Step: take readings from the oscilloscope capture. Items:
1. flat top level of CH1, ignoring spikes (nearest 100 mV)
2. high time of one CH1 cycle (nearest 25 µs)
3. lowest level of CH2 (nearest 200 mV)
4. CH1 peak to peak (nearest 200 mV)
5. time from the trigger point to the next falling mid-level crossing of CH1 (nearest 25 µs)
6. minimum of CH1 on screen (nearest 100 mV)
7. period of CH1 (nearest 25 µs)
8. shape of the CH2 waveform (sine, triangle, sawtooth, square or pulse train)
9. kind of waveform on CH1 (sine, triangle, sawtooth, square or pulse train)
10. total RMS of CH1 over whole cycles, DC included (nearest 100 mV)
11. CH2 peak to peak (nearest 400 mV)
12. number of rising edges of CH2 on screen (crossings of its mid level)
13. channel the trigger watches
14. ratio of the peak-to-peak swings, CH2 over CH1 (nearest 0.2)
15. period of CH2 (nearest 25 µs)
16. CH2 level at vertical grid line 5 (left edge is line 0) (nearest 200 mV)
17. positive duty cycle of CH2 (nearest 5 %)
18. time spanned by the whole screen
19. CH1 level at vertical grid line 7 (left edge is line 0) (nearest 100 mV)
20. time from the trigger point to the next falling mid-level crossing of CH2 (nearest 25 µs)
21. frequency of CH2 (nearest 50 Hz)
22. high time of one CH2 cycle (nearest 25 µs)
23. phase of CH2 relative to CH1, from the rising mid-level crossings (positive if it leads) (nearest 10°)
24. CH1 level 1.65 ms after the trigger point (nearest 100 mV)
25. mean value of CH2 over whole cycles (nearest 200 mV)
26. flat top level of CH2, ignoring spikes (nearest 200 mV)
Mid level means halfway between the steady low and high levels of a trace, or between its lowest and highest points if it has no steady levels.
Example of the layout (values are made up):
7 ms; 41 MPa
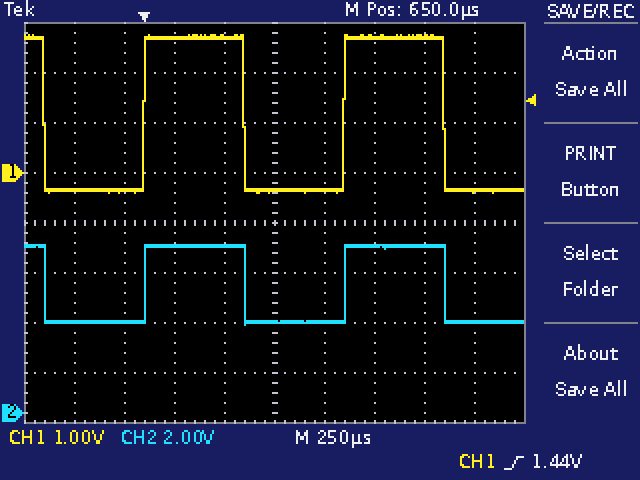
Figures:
2.7 V; 500 µs; 3.6 V; 3.2 V; 500 µs; -400 mV; 1.000 ms; square; square; 1.9 V; 3.2 V; 2; CH1; 1.0; 1.000 ms; 3.6 V; 50 %; 2.5 ms; 2.7 V; 500 µs; 1.00 kHz; 500 µs; 0°; -400 mV; 5.2 V; 6.6 V
